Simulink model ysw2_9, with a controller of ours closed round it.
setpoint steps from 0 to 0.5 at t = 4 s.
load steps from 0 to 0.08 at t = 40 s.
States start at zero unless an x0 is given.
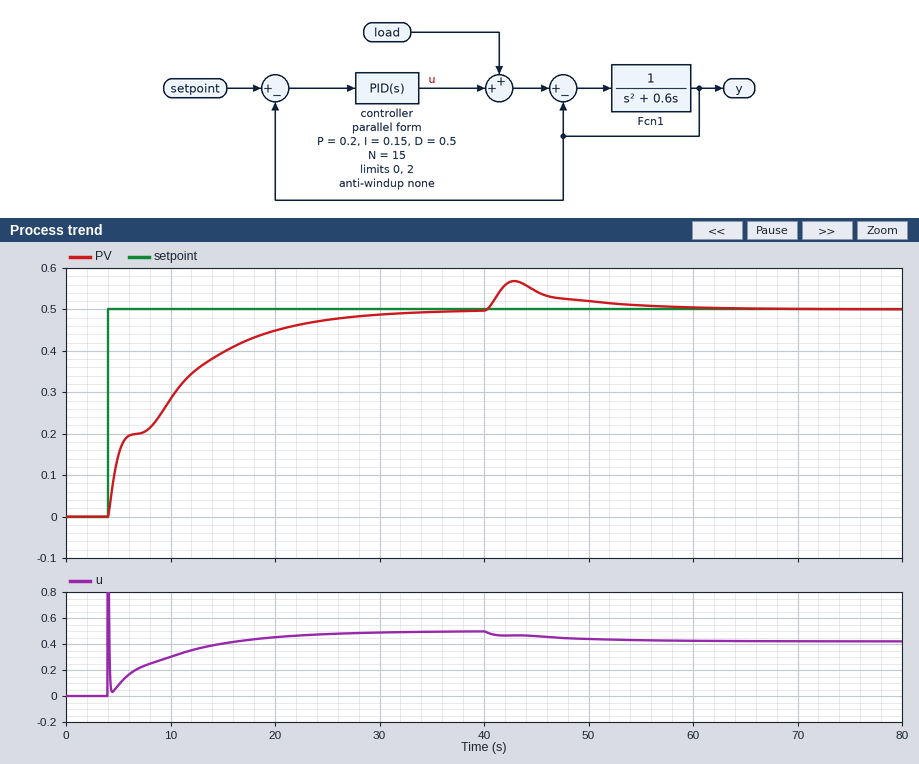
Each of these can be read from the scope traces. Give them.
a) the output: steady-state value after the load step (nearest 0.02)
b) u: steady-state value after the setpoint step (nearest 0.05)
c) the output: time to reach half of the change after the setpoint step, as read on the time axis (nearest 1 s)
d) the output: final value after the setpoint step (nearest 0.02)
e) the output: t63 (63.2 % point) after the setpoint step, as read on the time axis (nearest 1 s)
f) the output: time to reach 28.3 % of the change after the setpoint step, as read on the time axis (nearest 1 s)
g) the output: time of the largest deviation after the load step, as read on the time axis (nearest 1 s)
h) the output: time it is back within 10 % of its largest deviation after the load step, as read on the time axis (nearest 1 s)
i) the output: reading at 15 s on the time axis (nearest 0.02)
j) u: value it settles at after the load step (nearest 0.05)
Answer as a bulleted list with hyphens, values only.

- 0.50
- 0.50
- 9 s
- 0.50
- 11 s
- 5 s
- 43 s
- 57 s
- 0.40
- 0.40
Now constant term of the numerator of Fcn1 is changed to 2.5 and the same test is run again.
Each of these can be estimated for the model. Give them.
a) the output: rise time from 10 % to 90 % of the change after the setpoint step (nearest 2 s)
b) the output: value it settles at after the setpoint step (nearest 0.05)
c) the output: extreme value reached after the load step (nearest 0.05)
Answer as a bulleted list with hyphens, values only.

- 16 s
- 0.50
- 0.55
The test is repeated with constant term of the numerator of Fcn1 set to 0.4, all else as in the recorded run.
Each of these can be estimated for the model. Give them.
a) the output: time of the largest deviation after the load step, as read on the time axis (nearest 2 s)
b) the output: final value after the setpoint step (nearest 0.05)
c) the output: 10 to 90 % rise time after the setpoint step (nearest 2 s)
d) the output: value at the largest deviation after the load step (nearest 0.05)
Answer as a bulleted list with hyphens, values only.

- 44 s
- 0.50
- 14 s
- 0.55
